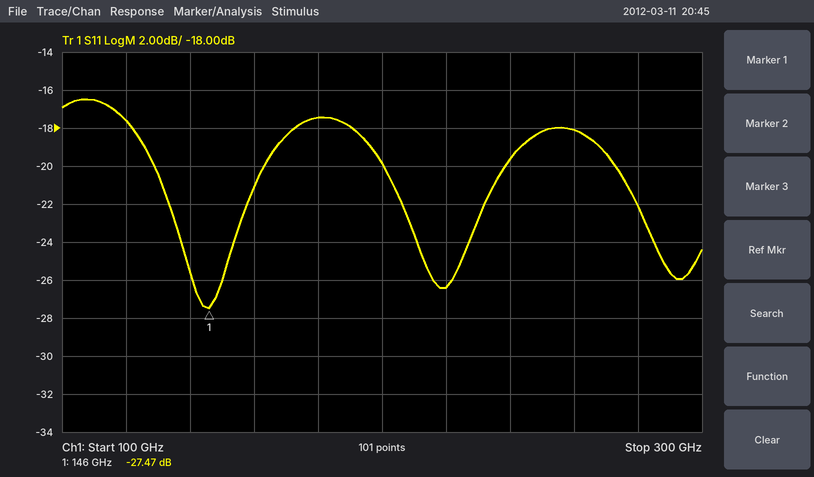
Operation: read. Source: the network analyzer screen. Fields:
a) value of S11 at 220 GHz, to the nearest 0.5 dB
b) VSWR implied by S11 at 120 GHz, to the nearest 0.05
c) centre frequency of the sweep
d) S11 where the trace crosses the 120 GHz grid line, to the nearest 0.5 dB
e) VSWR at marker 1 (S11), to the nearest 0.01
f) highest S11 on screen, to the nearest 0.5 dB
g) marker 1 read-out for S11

-26.5 dB
1.30
200 GHz
-17.5 dB
1.09
-16.5 dB
-27.47 dB
